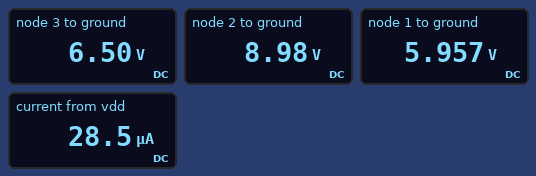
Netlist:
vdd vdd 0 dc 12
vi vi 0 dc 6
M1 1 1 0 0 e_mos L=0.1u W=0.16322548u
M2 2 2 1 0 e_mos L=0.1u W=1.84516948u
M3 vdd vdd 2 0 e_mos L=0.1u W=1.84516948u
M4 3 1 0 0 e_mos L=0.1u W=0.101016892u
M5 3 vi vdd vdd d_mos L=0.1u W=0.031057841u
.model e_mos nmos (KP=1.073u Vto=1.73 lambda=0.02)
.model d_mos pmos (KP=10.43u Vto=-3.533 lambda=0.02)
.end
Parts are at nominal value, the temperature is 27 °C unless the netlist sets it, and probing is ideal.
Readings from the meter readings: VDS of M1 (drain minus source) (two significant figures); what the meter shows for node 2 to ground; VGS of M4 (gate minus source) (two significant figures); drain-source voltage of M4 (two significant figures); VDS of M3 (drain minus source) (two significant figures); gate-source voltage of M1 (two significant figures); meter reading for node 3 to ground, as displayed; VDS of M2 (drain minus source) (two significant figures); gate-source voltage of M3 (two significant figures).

6.0 V
8.98 V
6.0 V
6.5 V
3.0 V
6.0 V
6.50 V
3.0 V
3.0 V
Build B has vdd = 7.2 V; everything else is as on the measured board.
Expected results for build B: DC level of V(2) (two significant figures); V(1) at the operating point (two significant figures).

5.1 V
3.0 V
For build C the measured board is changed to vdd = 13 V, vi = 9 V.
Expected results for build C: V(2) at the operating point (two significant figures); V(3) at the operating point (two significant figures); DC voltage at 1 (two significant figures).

9.8 V
85 mV
6.6 V
